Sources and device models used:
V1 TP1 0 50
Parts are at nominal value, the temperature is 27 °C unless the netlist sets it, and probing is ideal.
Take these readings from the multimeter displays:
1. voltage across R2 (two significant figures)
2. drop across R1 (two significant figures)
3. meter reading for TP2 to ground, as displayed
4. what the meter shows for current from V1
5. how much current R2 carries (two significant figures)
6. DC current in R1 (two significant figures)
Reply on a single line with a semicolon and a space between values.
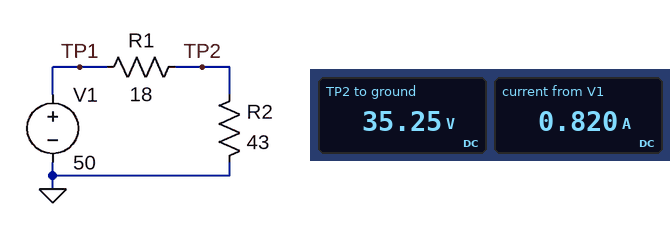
35 V; 15 V; 35.25 V; 0.820 A; 820 mA; 820 mA
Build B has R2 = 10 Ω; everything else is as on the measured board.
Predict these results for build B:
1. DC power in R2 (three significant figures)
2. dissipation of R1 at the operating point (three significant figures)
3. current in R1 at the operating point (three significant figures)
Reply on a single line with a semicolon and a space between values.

31.9 W; 57.4 W; 1.79 A
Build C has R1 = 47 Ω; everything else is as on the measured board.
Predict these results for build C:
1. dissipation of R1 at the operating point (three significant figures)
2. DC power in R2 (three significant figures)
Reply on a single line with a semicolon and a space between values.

14.5 W; 13.3 W
